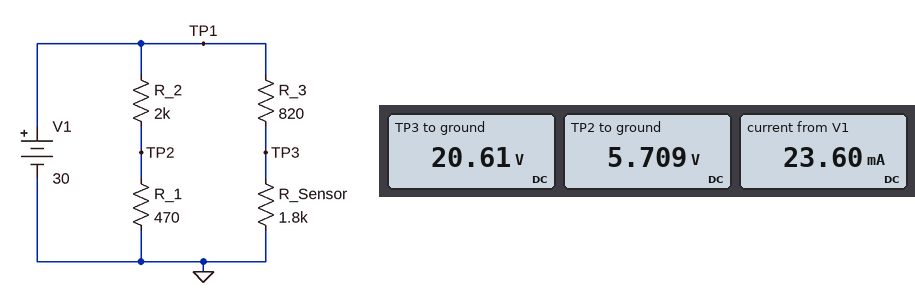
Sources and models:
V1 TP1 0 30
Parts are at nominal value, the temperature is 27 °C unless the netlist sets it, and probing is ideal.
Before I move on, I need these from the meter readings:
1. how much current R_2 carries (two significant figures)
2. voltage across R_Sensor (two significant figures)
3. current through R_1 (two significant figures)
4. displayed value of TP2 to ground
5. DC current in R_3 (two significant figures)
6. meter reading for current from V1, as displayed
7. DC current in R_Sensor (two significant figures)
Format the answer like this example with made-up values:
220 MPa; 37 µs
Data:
12 mA; 21 V; 12 mA; 5.709 V; 11 mA; 23.60 mA; 11 mA
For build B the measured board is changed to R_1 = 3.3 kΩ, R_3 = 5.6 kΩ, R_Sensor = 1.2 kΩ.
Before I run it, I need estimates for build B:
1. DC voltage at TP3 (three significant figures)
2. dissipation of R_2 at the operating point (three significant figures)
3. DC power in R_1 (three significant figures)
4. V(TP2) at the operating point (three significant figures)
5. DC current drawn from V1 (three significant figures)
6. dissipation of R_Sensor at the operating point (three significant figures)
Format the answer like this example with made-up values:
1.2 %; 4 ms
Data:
5.29 V; 64.1 mW; 106 mW; 18.7 V; 10.1 mA; 23.4 mW
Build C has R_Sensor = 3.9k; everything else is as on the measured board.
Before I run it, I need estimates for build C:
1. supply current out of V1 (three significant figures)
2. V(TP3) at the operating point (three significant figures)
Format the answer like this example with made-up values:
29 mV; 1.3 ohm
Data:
18.5 mA; 24.8 V
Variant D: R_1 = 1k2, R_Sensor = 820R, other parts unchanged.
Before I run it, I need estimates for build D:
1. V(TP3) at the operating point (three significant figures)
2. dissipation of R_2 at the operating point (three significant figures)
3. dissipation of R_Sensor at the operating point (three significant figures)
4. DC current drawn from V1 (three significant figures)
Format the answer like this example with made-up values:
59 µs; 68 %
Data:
15.0 V; 176 mW; 274 mW; 27.7 mA
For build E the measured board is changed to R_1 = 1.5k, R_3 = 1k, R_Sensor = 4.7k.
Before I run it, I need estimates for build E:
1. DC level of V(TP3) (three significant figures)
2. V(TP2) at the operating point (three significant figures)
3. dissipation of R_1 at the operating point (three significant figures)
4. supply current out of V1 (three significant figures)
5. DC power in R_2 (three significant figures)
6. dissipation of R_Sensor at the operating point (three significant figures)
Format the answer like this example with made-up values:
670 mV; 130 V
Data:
24.7 V; 12.9 V; 110 mW; 13.8 mA; 147 mW; 130 mW
